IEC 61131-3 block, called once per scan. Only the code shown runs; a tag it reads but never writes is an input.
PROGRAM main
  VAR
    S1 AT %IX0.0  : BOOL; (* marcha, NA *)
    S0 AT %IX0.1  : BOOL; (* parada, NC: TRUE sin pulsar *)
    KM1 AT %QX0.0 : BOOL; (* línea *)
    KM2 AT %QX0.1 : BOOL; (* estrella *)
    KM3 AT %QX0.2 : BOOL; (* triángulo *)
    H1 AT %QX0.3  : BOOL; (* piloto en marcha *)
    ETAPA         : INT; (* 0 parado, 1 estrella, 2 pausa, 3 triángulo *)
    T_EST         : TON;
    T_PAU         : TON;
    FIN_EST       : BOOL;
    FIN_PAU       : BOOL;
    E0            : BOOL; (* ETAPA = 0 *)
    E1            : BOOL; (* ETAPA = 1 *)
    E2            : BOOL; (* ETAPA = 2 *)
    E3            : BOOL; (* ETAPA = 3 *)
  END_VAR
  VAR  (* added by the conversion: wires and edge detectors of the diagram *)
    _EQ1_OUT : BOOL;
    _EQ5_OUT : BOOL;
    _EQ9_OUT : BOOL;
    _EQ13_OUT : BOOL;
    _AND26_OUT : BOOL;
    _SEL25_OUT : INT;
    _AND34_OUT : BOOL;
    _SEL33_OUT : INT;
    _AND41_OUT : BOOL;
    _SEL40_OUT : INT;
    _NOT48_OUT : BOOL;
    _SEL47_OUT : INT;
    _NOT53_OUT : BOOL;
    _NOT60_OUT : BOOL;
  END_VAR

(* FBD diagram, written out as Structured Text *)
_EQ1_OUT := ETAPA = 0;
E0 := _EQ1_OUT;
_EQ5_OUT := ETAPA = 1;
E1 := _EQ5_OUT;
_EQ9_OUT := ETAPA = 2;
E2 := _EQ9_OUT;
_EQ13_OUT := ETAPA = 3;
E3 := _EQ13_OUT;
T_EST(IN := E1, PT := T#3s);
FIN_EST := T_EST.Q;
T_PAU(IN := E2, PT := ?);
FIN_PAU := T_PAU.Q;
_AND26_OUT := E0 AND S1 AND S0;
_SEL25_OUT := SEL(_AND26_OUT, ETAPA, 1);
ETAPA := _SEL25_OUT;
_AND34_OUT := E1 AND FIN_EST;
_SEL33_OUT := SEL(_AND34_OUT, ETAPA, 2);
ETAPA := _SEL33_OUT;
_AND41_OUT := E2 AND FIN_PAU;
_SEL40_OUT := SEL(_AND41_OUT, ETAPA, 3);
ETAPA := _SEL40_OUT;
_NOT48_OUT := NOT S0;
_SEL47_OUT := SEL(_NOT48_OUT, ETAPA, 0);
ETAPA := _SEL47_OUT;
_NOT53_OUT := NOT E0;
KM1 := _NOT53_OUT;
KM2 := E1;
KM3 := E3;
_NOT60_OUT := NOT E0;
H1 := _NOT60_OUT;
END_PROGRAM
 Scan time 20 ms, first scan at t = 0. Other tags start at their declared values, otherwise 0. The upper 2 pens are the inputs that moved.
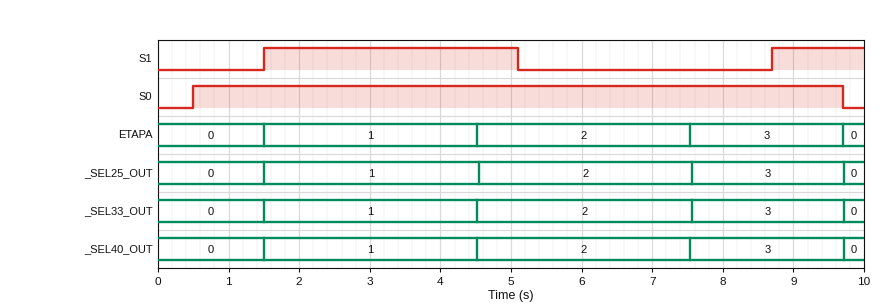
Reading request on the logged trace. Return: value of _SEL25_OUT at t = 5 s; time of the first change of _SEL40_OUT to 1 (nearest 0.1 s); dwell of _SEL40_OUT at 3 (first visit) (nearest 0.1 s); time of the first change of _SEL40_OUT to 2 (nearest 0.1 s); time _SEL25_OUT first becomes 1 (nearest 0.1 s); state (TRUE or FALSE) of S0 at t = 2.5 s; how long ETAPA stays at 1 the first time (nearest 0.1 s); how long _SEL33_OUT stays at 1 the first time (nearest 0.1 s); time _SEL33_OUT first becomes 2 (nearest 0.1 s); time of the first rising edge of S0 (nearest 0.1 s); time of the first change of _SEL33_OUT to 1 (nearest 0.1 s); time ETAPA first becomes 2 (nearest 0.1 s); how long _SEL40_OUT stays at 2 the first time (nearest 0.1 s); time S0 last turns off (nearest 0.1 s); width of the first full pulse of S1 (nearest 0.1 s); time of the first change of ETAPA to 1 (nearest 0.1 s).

2
1.5 s
2.2 s
4.5 s
1.5 s
TRUE
3.0 s
3.0 s
4.5 s
0.5 s
1.5 s
4.5 s
3.0 s
9.7 s
3.6 s
1.5 s
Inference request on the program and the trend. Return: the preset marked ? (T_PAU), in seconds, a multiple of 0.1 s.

3.0 s
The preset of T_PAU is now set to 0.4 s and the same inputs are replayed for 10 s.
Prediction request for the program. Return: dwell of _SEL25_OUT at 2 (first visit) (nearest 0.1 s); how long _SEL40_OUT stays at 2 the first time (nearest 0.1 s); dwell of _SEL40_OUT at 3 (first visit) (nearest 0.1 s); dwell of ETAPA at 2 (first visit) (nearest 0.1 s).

0.4 s
0.4 s
4.8 s
0.4 s
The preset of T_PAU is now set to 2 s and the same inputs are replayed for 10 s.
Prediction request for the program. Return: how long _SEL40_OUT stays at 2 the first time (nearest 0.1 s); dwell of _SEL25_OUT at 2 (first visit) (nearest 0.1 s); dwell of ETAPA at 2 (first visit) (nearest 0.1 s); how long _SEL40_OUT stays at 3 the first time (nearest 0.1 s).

2.0 s
2.0 s
2.0 s
3.2 s
